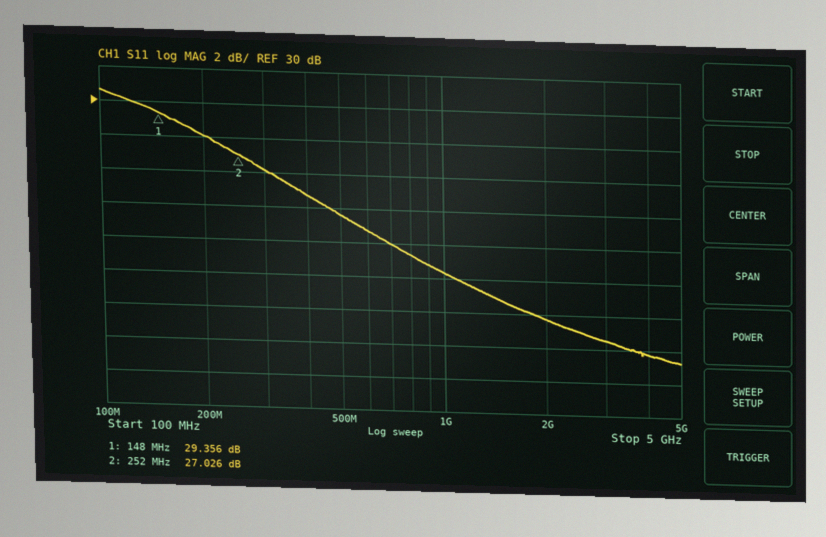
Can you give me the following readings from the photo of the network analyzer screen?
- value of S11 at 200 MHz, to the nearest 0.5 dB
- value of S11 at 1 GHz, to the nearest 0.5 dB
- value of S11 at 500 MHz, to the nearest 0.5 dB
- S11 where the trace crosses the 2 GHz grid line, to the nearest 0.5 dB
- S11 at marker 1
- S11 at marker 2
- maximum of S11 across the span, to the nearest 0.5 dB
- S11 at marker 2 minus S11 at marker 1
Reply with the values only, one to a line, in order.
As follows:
28.0 dB
20.5 dB
23.5 dB
17.5 dB
29.356 dB
27.026 dB
30.5 dB
-2.330 dB
